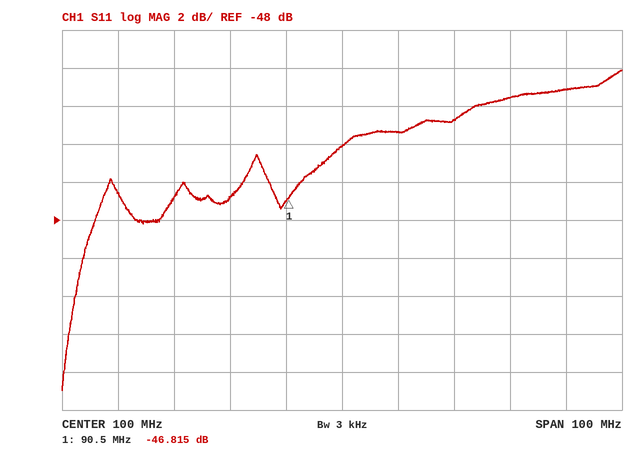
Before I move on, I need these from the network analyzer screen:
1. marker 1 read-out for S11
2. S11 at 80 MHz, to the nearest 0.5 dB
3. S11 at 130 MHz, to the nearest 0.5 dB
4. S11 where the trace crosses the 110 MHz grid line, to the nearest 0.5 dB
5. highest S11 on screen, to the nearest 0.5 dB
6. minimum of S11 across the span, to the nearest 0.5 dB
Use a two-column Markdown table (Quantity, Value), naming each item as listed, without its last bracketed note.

| Quantity | Value |
|---|---|
| marker 1 read-out for S11 | -46.815 dB |
| S11 at 80 MHz, to the nearest 0.5 dB | -47.0 dB |
| S11 at 130 MHz, to the nearest 0.5 dB | -41.5 dB |
| S11 where the trace crosses the 110 MHz grid line, to the nearest 0.5 dB | -43.5 dB |
| highest S11 on screen, to the nearest 0.5 dB | -40.0 dB |
| minimum of S11 across the span, to the nearest 0.5 dB | -57.0 dB |
